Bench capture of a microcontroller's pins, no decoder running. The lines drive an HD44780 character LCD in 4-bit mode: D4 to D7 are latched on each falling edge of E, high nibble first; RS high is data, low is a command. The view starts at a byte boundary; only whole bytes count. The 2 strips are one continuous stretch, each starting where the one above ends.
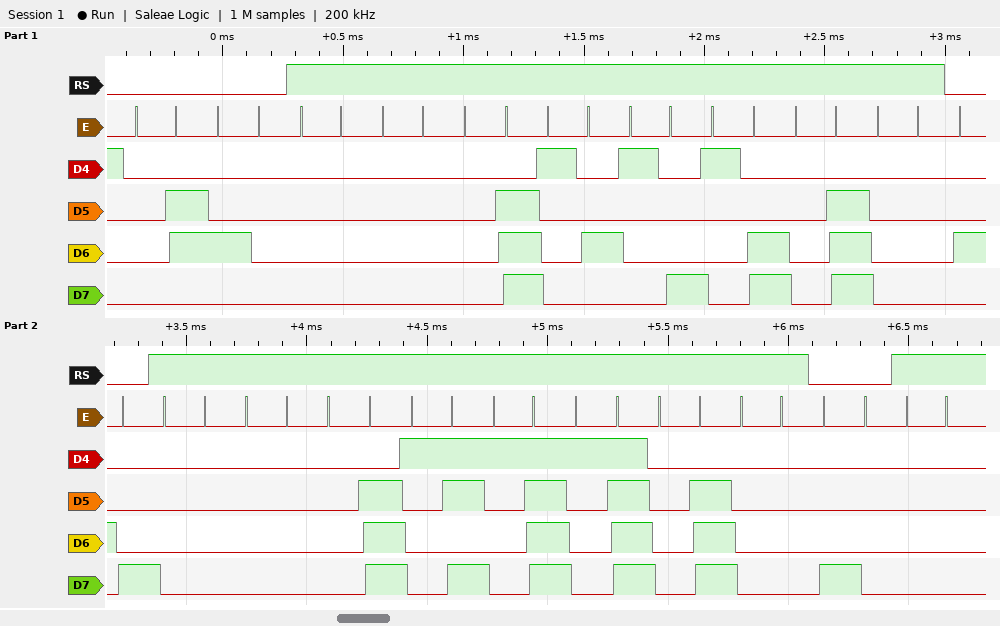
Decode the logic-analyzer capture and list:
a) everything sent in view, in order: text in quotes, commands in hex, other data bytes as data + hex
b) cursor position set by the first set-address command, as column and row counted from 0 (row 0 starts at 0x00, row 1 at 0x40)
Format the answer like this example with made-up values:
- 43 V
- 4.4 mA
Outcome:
- 0x06 0x40 data 00 00 0E 14 18 1C 0E 00 0x48 data 00 00 0E 1B 1F 1F 0E 00 0x80 data 00
- column 0, row 0
